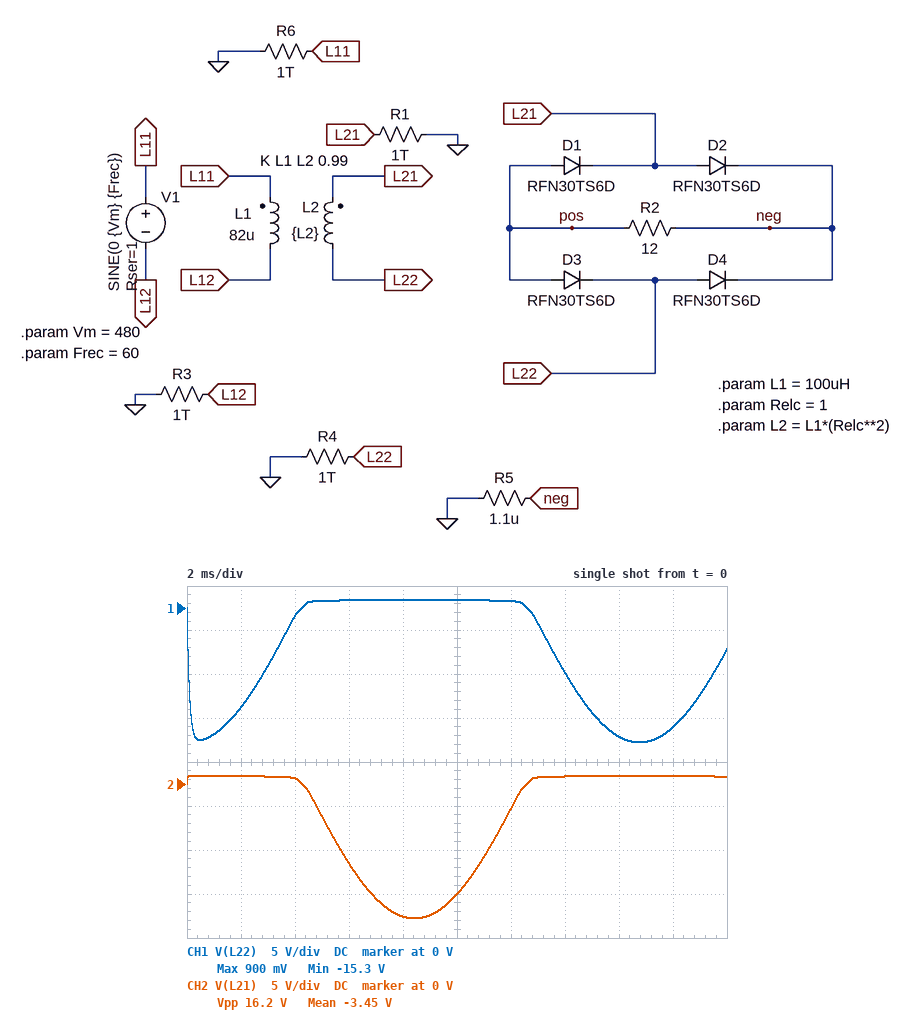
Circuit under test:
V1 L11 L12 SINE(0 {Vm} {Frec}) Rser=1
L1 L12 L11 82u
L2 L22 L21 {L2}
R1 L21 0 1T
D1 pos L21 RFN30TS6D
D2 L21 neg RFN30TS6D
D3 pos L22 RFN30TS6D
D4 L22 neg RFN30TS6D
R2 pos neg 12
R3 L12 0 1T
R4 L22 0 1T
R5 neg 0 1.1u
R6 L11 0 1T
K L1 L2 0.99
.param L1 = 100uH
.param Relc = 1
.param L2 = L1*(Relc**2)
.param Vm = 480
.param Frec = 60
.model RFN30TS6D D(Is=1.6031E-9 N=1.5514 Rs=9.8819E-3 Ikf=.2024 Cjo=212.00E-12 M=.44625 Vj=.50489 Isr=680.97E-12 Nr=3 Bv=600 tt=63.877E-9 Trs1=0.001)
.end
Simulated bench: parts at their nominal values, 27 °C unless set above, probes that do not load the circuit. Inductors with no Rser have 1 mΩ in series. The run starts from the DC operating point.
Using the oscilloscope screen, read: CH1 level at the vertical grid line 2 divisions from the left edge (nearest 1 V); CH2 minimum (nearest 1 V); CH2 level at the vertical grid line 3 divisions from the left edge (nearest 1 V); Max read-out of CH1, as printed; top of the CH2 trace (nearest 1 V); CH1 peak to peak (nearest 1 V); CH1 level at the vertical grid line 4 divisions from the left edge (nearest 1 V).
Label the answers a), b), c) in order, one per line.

a) -1 V
b) -15 V
c) -9 V
d) 900 mV
e) 1 V
f) 16 V
g) 1 V
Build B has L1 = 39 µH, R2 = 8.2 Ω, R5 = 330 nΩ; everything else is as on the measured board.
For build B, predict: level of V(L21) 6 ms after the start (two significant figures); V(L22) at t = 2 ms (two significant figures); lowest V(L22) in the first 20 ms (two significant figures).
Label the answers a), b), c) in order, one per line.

a) -6.1 V
b) -7.4 V
c) -10 V
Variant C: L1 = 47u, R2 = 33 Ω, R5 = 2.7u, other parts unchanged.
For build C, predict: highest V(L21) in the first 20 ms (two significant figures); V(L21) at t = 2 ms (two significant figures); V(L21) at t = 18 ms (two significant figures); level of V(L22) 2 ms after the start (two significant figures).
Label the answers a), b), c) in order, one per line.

a) 820 mV
b) 800 mV
c) 810 mV
d) -8.3 V
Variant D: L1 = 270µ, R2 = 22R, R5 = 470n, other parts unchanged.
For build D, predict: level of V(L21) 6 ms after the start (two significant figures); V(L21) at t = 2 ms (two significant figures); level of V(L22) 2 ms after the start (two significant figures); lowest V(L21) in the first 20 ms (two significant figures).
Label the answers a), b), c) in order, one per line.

a) -15 V
b) 900 mV
c) -22 V
d) -28 V
